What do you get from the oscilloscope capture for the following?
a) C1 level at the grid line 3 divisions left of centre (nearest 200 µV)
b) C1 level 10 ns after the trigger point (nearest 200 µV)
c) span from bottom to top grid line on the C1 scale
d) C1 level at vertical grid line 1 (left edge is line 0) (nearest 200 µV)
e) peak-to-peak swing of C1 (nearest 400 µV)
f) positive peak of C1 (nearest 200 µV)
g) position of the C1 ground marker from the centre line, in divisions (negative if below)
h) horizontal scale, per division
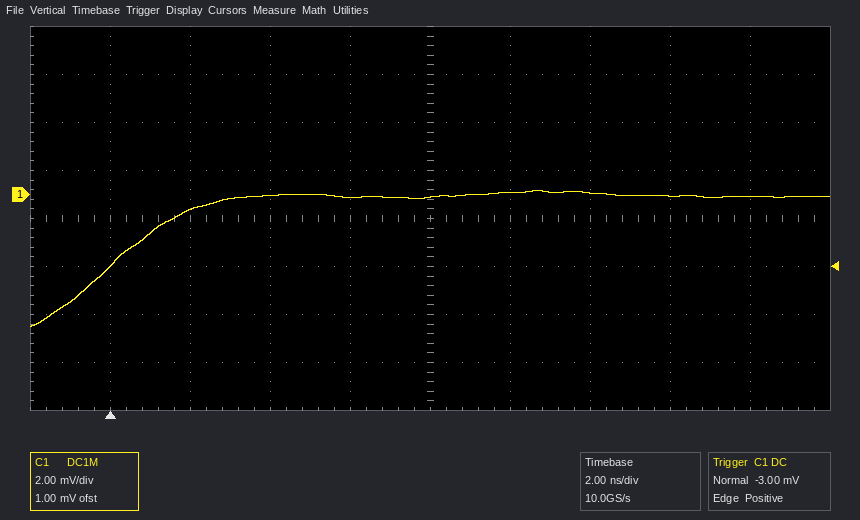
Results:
-600 µV
0.0 mV
16 mV
-3.0 mV
5.6 mV
200 µV
+0.5 div
2 ns
